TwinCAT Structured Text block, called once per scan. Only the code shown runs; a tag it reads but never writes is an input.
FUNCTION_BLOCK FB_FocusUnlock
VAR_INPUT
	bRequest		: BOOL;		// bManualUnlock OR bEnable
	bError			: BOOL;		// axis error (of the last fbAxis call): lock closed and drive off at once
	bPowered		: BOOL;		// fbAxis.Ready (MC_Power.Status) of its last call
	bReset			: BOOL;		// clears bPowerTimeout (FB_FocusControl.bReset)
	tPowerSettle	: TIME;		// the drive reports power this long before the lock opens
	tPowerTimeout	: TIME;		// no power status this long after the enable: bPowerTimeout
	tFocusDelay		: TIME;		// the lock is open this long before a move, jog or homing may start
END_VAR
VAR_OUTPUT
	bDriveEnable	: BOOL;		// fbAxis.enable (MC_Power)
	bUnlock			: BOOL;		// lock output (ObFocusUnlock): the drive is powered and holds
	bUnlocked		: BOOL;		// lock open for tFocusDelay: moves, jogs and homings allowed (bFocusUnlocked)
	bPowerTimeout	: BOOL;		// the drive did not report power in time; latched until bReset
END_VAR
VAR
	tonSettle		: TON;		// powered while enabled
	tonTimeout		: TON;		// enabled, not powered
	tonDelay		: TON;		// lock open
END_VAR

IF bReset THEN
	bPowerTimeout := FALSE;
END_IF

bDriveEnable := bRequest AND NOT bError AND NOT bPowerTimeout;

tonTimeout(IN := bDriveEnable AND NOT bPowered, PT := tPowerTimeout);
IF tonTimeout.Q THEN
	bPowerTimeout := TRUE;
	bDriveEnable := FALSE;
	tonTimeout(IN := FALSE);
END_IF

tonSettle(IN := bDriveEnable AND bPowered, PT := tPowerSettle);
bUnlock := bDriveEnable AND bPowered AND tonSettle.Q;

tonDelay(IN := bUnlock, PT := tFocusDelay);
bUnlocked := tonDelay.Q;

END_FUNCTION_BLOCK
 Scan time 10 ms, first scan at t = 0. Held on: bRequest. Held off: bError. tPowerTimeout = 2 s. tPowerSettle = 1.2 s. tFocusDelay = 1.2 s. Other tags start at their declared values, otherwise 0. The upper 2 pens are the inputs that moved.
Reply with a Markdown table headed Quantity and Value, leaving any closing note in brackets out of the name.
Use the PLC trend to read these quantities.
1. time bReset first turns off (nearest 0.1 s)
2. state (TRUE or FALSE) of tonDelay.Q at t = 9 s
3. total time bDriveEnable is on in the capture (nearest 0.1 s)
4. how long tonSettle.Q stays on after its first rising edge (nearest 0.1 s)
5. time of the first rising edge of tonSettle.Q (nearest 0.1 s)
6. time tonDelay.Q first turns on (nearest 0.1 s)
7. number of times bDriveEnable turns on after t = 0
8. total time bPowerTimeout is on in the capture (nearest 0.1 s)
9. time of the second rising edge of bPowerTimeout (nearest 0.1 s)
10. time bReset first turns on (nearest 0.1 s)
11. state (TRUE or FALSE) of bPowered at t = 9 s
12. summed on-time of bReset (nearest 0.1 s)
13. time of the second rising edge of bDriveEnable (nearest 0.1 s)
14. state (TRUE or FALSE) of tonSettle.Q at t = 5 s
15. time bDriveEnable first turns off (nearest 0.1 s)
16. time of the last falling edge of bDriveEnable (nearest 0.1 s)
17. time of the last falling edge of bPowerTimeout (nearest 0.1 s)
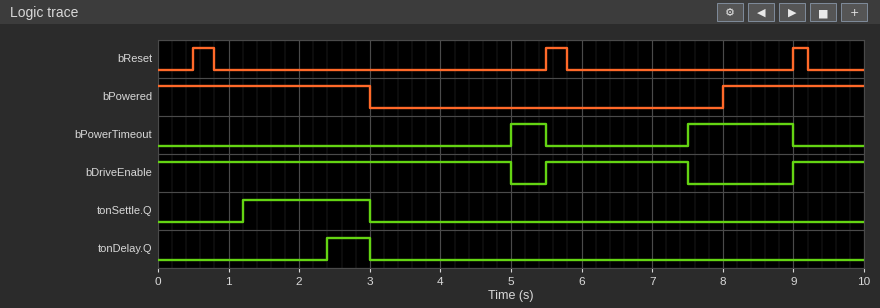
| Quantity | Value |
|---|---|
| time bReset first turns off | 0.8 s |
| state (TRUE or FALSE) of tonDelay.Q at t = 9 s | FALSE |
| total time bDriveEnable is on in the capture | 8.0 s |
| how long tonSettle.Q stays on after its first rising edge | 1.8 s |
| time of the first rising edge of tonSettle.Q | 1.2 s |
| time tonDelay.Q first turns on | 2.4 s |
| number of times bDriveEnable turns on after t = 0 | 2 |
| total time bPowerTimeout is on in the capture | 2.0 s |
| time of the second rising edge of bPowerTimeout | 7.5 s |
| time bReset first turns on | 0.5 s |
| state (TRUE or FALSE) of bPowered at t = 9 s | TRUE |
| summed on-time of bReset | 0.8 s |
| time of the second rising edge of bDriveEnable | 9.0 s |
| state (TRUE or FALSE) of tonSettle.Q at t = 5 s | FALSE |
| time bDriveEnable first turns off | 5.0 s |
| time of the last falling edge of bDriveEnable | 7.5 s |
| time of the last falling edge of bPowerTimeout | 9.0 s |
